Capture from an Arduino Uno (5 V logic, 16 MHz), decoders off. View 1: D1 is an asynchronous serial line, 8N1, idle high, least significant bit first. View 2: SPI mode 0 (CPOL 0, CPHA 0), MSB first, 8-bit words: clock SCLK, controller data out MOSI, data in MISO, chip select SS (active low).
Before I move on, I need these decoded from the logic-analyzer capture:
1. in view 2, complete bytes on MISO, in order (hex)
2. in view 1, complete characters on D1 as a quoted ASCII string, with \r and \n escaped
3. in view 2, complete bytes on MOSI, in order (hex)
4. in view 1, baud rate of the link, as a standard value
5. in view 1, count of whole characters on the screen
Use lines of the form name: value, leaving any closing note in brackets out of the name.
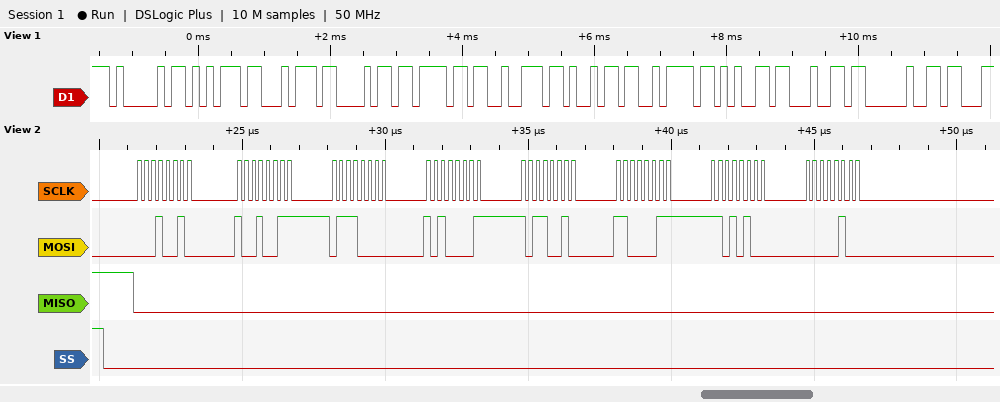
in view 2, complete bytes on MISO, in order: 0x00 0x00 0x00 0x00 0x00 0x00 0x00 0x00
in view 1, complete characters on D1 as a quoted ASCII string, with \r and \n escaped: "Authorized "
in view 2, complete bytes on MOSI, in order: 0x12 0x93 0x70 0xA1 0xB2 0xC3 0xD4 0x04
in view 1, baud rate of the link, as a standard value: 9600 baud
in view 1, count of whole characters on the screen: 11
